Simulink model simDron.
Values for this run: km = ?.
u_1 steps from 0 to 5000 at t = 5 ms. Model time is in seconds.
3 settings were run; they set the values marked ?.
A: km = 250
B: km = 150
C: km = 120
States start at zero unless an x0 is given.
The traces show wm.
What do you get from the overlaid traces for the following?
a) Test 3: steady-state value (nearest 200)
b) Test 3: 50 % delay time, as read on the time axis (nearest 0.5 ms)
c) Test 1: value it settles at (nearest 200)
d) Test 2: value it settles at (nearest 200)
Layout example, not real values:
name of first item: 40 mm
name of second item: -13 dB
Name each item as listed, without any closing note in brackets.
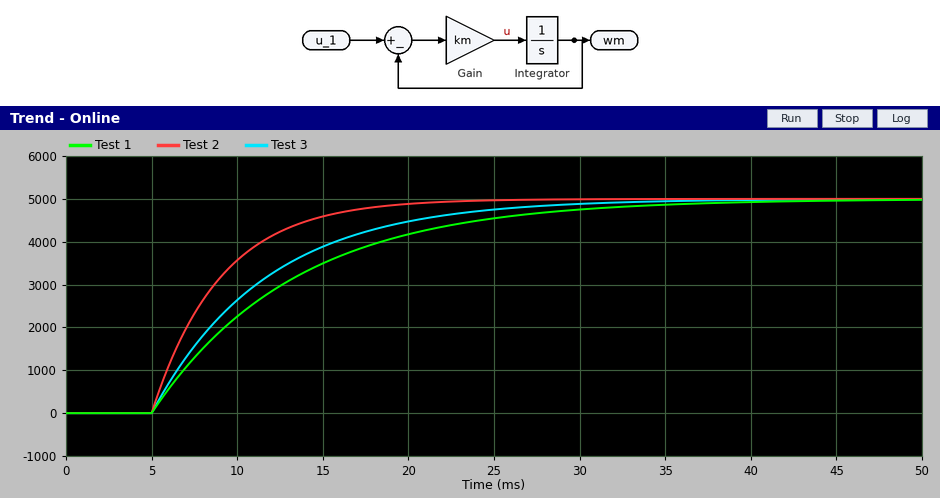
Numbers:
Test 3: steady-state value: 5000
Test 3: 50 % delay time, as read on the time axis: 9.5 ms
Test 1: value it settles at: 5000
Test 2: value it settles at: 5000
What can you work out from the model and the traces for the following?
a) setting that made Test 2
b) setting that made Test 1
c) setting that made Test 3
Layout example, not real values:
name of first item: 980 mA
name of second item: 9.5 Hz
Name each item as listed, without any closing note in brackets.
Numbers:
setting that made Test 2: A
setting that made Test 1: C
setting that made Test 3: B
